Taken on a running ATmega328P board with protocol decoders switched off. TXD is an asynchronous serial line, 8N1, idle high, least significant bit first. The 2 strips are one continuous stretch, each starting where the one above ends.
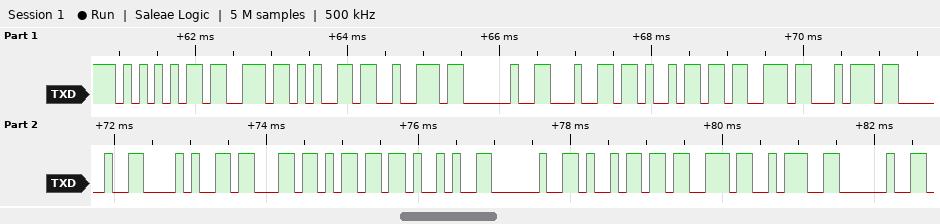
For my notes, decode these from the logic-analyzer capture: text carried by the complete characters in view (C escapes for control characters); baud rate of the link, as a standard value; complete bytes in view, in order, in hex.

"User dist (cm) is: "
9600 baud
55 73 65 72 20 64 69 73 74 20 28 63 6D 29 20 69 73 3A 20
